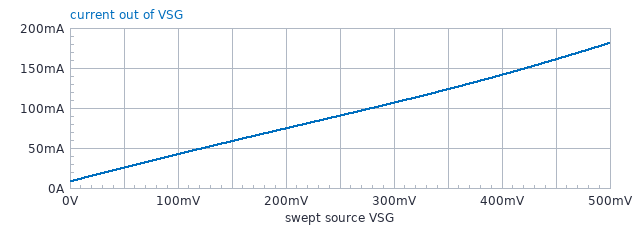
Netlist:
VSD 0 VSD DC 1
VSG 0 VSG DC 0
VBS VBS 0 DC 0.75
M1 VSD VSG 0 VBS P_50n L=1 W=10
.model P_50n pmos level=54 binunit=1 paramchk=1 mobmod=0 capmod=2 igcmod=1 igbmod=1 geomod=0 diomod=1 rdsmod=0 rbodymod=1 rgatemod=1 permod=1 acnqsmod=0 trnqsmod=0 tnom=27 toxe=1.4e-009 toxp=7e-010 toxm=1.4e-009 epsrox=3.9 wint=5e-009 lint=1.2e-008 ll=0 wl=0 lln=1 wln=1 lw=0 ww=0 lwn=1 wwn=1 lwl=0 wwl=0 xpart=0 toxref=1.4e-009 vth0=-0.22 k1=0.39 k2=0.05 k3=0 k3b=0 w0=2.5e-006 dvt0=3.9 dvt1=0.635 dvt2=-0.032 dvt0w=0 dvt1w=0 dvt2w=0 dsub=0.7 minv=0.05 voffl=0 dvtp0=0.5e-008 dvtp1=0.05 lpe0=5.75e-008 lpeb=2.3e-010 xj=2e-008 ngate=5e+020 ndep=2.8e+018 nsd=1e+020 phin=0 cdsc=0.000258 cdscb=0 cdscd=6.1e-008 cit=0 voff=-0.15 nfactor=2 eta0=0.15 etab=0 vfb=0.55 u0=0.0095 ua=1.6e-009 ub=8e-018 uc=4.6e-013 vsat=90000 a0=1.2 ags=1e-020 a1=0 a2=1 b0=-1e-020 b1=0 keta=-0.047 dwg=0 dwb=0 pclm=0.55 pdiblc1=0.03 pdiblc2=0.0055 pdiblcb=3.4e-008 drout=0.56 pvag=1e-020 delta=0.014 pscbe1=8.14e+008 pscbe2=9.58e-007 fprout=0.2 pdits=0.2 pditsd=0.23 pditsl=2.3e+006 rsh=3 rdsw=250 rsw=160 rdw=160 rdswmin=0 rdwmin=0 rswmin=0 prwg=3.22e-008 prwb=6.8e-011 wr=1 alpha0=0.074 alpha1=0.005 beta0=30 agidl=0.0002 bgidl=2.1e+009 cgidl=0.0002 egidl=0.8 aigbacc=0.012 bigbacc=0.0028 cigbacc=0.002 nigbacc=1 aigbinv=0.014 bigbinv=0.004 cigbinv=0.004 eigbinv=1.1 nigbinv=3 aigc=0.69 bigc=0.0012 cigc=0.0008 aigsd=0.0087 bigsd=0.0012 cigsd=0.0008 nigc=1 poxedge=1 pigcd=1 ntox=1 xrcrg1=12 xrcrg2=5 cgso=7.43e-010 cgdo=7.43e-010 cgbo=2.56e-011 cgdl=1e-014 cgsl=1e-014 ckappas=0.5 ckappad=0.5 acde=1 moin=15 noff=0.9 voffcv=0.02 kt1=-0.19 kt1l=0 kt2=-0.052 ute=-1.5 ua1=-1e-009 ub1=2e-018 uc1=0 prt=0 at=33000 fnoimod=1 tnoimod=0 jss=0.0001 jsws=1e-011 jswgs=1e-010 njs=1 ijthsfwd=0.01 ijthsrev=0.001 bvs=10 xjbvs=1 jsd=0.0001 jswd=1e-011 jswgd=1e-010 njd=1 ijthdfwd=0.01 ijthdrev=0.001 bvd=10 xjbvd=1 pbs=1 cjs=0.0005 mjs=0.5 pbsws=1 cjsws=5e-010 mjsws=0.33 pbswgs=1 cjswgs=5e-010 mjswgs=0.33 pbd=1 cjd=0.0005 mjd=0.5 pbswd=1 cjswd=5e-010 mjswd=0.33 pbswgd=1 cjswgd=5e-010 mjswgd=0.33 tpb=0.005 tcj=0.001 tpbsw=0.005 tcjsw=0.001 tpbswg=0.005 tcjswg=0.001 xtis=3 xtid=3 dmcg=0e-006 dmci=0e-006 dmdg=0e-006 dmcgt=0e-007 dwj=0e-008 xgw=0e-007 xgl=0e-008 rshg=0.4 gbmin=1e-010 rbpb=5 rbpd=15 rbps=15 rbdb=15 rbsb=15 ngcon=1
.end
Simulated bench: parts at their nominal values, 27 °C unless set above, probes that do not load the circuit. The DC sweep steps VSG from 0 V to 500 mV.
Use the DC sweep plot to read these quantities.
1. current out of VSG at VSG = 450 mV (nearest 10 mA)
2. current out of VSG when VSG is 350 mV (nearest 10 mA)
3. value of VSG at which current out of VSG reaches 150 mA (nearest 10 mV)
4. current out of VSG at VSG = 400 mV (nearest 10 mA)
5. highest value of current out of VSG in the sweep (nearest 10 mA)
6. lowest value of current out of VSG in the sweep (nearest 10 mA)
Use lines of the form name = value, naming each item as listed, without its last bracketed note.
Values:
current out of VSG at VSG = 450 mV = 160 mA
current out of VSG when VSG is 350 mV = 120 mA
value of VSG at which current out of VSG reaches 150 mA = 420 mV
current out of VSG at VSG = 400 mV = 140 mA
highest value of current out of VSG in the sweep = 180 mA
lowest value of current out of VSG in the sweep = 10 mA
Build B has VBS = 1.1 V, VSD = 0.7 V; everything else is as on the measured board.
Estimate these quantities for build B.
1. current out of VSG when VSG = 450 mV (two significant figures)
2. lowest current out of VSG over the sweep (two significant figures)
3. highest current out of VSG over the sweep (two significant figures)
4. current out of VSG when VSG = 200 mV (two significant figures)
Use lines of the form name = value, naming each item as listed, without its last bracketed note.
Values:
current out of VSG when VSG = 450 mV = 220 mA
lowest current out of VSG over the sweep = 110 mA
highest current out of VSG over the sweep = 240 mA
current out of VSG when VSG = 200 mV = 160 mA
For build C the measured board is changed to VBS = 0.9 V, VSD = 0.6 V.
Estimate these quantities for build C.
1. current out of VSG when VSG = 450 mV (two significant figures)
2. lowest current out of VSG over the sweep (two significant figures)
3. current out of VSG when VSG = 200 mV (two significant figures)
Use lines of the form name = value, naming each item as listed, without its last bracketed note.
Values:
current out of VSG when VSG = 450 mV = 200 mA
lowest current out of VSG over the sweep = 96 mA
current out of VSG when VSG = 200 mV = 140 mA
